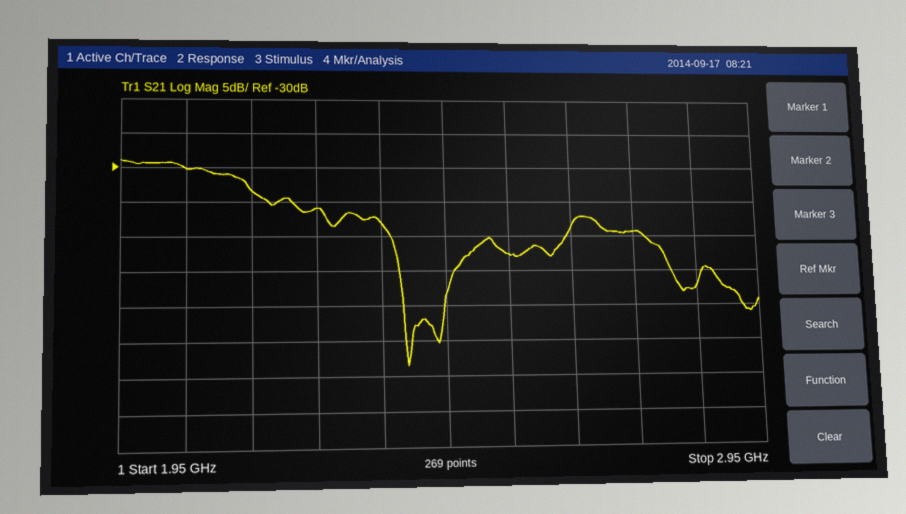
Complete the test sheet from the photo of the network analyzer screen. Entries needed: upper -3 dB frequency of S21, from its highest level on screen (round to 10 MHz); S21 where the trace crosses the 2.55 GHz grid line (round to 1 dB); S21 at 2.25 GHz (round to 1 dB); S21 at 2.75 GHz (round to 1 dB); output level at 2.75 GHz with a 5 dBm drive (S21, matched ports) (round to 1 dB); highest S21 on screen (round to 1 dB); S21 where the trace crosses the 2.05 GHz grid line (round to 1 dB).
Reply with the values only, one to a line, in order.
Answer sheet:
2.14 GHz
-43 dB
-36 dB
-39 dB
-34 dBm
-29 dB
-30 dB
